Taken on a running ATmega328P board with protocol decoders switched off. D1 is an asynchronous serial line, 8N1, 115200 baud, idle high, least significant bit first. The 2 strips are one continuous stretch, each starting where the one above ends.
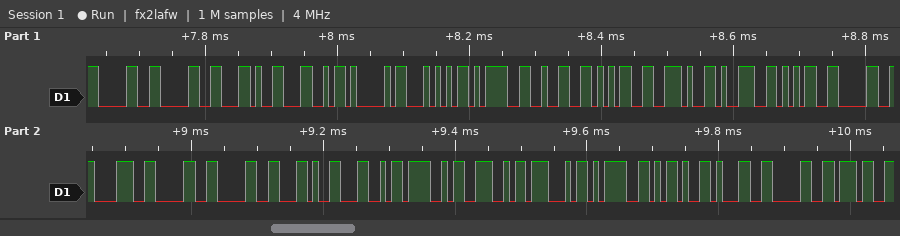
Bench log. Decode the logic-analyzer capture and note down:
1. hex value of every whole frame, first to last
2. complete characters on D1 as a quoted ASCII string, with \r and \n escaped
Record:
30 30 2C 4C 41 54 3D 32 35 2E 39 35 30 38 30 30 2C 4C 4F 4E 47 3D 2D 31 30 37
"00,LAT=25.950800,LONG=-107"
